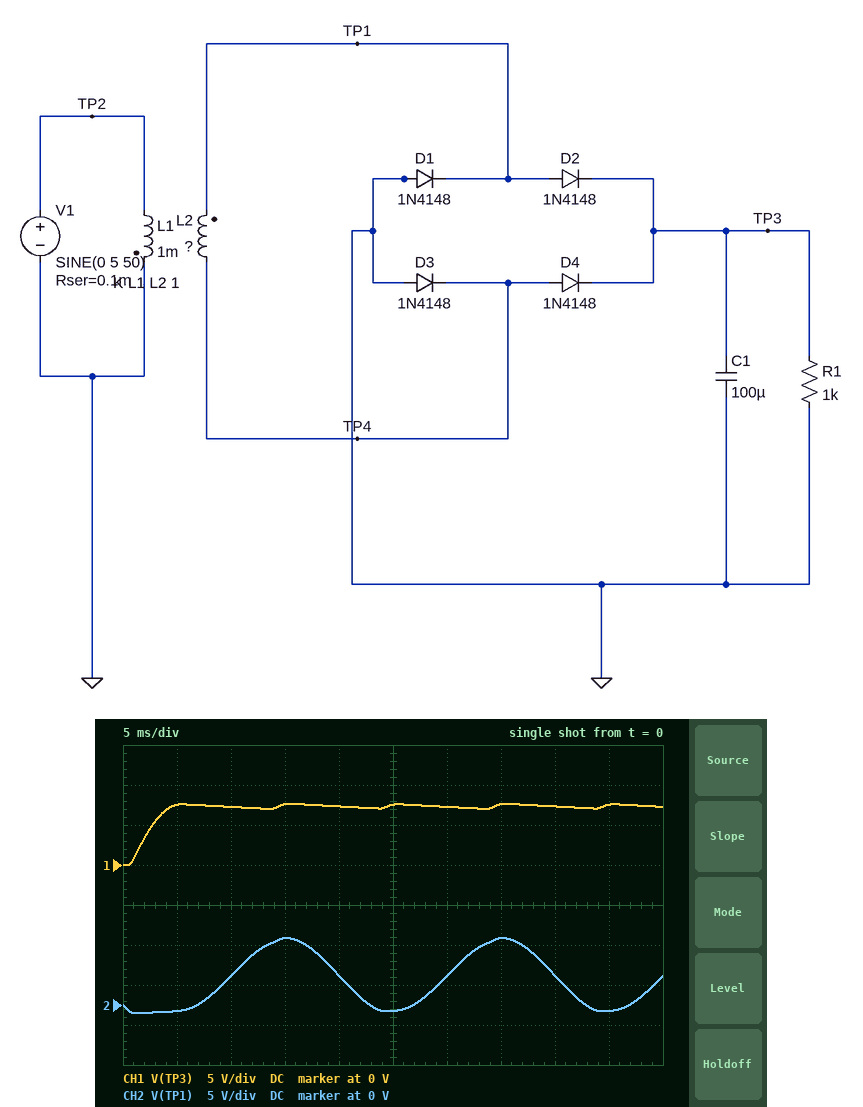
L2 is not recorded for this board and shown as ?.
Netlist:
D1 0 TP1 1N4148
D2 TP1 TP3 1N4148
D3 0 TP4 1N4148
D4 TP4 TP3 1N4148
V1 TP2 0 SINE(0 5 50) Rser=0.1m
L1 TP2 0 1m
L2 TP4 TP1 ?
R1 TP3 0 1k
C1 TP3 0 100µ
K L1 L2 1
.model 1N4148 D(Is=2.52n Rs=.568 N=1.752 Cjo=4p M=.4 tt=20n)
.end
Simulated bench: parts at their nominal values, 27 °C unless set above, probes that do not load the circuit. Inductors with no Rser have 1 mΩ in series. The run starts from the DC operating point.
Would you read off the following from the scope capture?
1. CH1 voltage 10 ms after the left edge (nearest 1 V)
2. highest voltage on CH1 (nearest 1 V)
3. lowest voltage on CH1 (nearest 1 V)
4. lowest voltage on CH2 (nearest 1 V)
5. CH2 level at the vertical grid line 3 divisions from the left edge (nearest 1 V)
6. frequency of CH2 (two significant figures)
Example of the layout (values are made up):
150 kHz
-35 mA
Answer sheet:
7 V
8 V
0 V
-1 V
8 V
50 Hz
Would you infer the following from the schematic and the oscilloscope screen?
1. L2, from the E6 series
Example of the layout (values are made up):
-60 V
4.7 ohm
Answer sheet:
3.3 mH
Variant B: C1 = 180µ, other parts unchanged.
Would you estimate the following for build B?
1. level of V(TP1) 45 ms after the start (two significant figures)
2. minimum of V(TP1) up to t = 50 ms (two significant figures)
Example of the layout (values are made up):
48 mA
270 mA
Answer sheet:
-790 mV
-1.1 V
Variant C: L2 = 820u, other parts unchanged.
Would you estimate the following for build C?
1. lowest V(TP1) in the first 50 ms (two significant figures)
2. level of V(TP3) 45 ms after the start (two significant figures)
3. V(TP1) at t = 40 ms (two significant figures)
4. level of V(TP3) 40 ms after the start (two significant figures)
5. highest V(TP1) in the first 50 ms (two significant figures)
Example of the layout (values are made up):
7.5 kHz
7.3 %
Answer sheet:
-870 mV
3.1 V
1.5 V
3.0 V
3.8 V
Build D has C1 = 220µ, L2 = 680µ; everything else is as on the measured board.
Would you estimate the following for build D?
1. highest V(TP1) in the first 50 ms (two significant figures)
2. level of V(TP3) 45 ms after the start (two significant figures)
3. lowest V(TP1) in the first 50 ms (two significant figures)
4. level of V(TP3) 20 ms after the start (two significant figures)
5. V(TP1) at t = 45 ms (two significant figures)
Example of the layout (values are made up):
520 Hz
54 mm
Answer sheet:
3.4 V
2.7 V
-950 mV
2.6 V
-720 mV
